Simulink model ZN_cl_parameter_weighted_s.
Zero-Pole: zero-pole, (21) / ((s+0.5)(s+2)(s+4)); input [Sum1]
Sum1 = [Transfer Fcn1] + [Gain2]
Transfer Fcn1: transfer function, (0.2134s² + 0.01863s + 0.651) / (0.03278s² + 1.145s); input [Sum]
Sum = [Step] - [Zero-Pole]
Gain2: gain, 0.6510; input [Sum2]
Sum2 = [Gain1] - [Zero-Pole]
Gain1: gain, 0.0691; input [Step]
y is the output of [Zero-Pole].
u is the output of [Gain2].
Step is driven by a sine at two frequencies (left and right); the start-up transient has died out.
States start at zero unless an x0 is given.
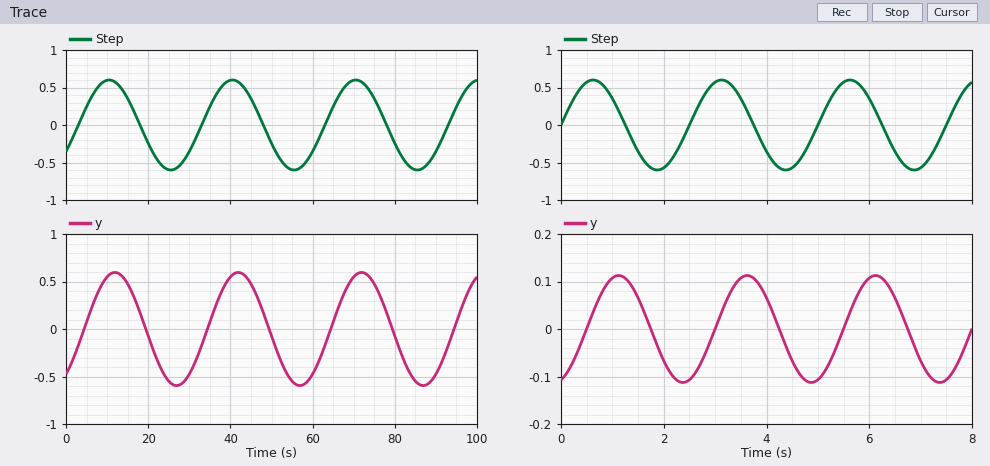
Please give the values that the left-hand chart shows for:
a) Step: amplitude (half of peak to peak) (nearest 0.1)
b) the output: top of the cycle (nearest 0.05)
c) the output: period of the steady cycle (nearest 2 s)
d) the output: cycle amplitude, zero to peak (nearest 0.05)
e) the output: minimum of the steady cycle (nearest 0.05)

0.6
0.60
30 s
0.60
-0.60
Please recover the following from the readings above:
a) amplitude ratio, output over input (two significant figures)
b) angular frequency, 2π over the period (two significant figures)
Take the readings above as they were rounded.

1.0
0.21 rad/s
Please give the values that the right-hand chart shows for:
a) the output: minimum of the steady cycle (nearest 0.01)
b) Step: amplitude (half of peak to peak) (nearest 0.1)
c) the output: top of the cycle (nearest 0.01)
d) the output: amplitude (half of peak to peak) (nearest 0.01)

-0.11
0.6
0.11
0.11
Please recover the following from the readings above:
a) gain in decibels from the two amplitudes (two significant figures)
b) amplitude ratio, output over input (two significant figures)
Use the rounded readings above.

-15 dB
0.18
